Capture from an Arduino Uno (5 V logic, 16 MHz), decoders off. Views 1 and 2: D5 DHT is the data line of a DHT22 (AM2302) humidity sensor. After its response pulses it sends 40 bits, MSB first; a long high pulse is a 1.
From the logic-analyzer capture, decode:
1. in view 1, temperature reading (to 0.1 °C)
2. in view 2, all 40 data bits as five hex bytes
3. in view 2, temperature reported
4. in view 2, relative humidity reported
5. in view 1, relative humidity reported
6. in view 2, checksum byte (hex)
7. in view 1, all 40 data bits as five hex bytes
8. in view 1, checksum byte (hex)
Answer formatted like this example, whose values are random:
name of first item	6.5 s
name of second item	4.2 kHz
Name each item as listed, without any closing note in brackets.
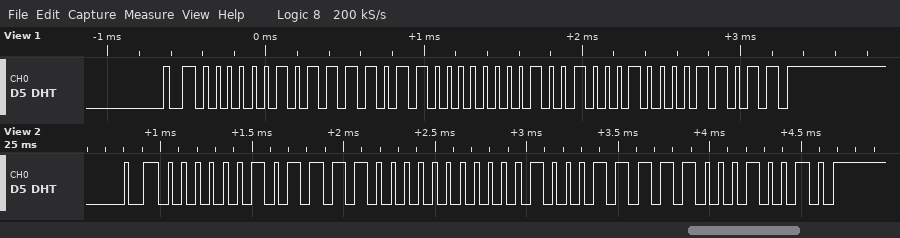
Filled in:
in view 1, temperature reading	29.0 °C
in view 2, all 40 data bits as five hex bytes	02 F0 01 1F 12
in view 2, temperature reported	28.7 °C
in view 2, relative humidity reported	75.2 %
in view 1, relative humidity reported	75.8 %
in view 2, checksum byte	0x12
in view 1, all 40 data bits as five hex bytes	02 F6 01 22 1B
in view 1, checksum byte	0x1B
